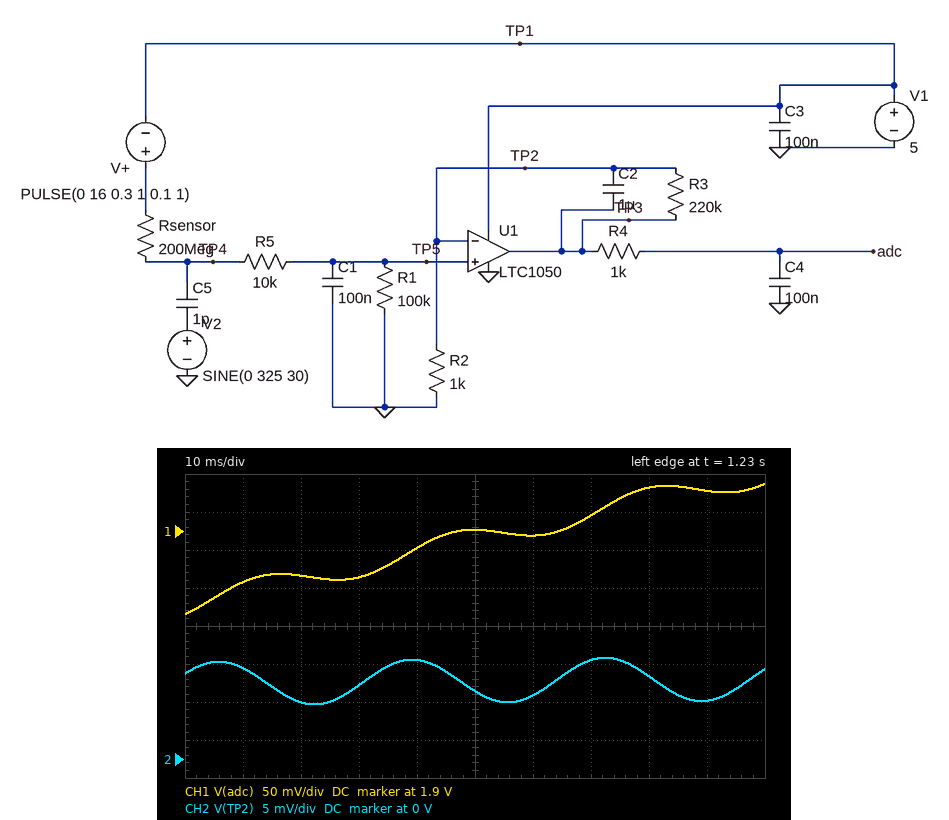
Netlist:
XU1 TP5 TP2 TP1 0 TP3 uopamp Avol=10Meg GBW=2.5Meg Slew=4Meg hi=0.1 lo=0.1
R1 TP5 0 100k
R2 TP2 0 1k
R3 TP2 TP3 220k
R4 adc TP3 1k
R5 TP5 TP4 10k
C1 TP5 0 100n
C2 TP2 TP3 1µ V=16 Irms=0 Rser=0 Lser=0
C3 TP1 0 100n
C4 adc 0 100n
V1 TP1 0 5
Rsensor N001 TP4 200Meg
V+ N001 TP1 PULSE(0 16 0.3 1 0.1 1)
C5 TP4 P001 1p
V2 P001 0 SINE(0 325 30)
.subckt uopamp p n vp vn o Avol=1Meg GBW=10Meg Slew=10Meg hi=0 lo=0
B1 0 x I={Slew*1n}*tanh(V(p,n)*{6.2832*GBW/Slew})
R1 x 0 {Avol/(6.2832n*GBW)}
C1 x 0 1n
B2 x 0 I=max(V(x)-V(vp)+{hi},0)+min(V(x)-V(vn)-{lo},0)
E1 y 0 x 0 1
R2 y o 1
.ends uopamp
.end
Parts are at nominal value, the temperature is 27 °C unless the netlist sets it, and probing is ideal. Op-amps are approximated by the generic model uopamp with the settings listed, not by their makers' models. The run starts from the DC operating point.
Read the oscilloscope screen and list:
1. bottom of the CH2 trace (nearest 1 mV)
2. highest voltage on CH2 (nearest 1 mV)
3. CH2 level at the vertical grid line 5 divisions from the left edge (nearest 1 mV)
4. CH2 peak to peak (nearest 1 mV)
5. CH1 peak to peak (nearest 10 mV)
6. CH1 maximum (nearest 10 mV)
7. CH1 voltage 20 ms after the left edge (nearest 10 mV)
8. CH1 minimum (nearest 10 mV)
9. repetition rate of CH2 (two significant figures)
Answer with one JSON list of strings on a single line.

["7 mV", "13 mV", "9 mV", "6 mV", "170 mV", "1.96 V", "1.84 V", "1.79 V", "30 Hz"]
